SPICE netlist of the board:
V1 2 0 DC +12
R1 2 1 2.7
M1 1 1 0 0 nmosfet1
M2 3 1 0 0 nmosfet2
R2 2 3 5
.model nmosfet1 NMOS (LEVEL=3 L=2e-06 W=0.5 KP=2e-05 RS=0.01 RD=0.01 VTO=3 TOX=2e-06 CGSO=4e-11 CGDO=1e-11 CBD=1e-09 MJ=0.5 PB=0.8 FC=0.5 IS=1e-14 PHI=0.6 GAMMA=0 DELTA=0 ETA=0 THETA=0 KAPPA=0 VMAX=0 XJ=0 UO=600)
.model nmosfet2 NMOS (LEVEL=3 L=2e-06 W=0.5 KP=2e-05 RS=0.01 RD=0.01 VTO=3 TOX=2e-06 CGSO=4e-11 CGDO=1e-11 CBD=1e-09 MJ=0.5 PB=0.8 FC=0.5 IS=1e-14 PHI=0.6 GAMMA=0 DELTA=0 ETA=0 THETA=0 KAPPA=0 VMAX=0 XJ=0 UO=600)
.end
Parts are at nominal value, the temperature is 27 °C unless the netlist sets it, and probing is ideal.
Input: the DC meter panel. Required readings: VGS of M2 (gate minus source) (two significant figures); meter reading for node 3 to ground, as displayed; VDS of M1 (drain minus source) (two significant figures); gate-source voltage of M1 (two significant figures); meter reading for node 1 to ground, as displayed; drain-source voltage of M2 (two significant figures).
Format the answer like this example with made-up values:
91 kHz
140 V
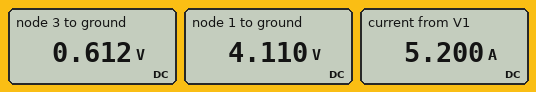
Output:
4.1 V
0.612 V
4.1 V
4.1 V
4.110 V
610 mV
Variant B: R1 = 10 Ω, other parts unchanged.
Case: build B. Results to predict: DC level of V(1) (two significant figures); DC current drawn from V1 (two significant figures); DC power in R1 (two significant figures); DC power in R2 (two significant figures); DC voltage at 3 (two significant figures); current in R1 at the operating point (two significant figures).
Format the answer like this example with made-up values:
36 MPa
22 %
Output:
3.6 V
1.7 A
7.1 W
3.5 W
7.8 V
840 mA
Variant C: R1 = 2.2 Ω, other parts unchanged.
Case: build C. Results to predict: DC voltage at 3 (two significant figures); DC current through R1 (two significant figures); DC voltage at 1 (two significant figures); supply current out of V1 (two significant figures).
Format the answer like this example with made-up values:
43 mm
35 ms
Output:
520 mV
3.5 A
4.2 V
5.8 A
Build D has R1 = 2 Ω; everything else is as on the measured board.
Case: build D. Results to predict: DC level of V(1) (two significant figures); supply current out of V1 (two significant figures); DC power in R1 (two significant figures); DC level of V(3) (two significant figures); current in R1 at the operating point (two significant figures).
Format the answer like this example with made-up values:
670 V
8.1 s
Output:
4.3 V
6.2 A
30 W
490 mV
3.9 A
